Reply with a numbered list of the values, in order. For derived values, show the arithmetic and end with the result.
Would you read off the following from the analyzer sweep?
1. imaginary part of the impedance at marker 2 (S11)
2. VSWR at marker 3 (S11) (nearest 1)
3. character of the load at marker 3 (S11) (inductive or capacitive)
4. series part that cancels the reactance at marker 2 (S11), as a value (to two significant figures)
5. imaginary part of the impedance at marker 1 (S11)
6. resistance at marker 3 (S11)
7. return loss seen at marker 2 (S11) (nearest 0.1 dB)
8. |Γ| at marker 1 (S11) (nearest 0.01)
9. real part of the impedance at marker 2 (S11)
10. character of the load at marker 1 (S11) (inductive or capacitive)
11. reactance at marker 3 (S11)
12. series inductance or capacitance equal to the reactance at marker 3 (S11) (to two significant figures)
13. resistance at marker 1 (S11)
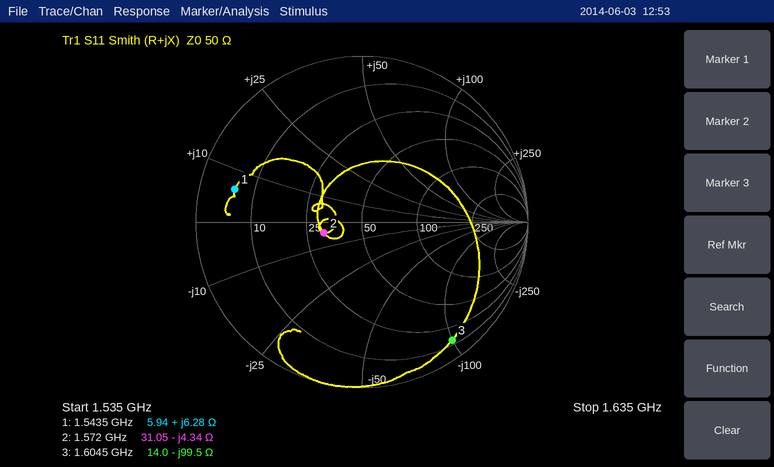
1. -4.34 Ω
2. 18
3. capacitive
4. L = 4.34 Ω/(2π × 1.572 GHz) ≈ 439 pH, so 440 pH to two significant figures
5. +6.28 Ω
6. 14.0 Ω
7. 12.4 dB
8. 0.79
9. 31.05 Ω
10. inductive
11. -99.5 Ω
12. C = 1/(2π × 1.6045 GHz × 99.5 Ω) ≈ 1.00 pF
13. 5.94 Ω
